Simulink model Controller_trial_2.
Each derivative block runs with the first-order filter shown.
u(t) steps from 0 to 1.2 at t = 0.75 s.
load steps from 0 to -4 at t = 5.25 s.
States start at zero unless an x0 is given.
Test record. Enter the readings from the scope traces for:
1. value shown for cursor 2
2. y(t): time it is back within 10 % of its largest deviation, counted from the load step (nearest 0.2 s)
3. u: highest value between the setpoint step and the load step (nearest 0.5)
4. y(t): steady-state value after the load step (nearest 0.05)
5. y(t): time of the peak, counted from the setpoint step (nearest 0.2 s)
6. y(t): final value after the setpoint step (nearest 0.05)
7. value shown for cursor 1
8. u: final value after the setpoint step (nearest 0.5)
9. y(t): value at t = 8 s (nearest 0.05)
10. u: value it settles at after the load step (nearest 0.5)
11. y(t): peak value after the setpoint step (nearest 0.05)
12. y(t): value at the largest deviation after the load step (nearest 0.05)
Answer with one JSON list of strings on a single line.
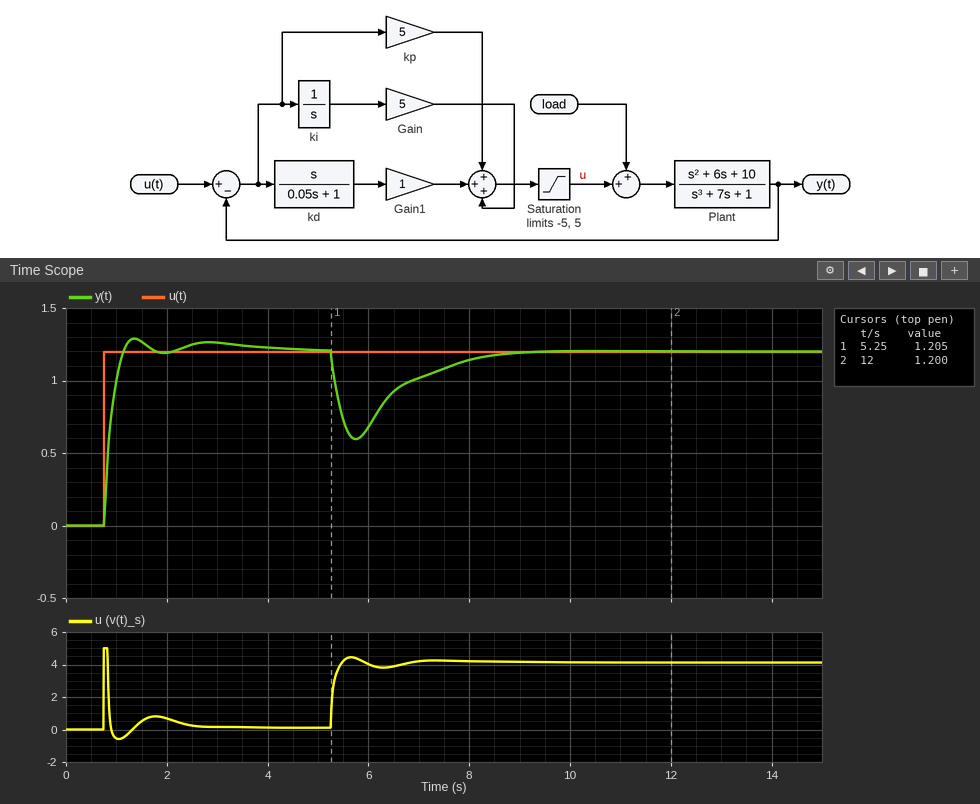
["1.200", "2.8 s", "5.0", "1.20", "0.6 s", "1.20", "1.205", "0.0", "1.15", "4.0", "1.30", "0.60"]
